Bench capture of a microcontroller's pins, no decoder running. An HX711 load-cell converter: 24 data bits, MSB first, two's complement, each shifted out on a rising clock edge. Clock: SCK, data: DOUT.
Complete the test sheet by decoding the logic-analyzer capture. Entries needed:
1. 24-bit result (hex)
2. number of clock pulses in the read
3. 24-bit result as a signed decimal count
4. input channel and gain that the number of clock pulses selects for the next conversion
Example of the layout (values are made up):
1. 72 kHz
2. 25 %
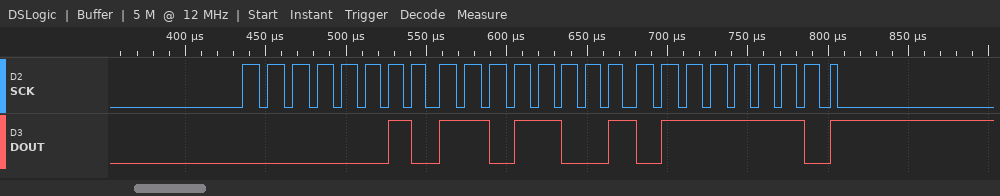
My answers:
1. 0x02D97E
2. 25
3. 186750
4. channel A, gain 128
